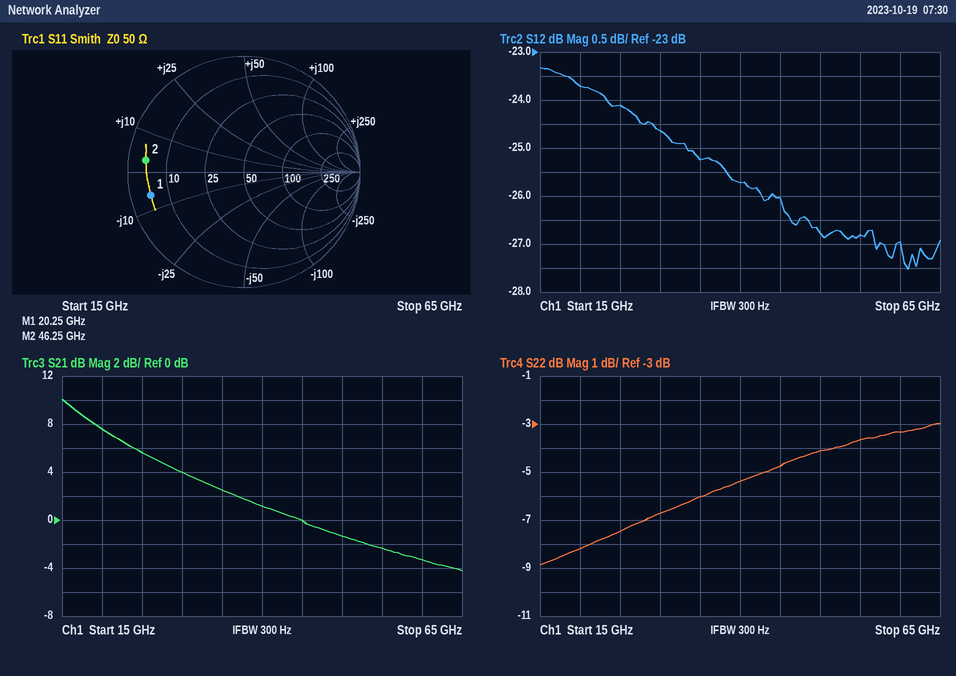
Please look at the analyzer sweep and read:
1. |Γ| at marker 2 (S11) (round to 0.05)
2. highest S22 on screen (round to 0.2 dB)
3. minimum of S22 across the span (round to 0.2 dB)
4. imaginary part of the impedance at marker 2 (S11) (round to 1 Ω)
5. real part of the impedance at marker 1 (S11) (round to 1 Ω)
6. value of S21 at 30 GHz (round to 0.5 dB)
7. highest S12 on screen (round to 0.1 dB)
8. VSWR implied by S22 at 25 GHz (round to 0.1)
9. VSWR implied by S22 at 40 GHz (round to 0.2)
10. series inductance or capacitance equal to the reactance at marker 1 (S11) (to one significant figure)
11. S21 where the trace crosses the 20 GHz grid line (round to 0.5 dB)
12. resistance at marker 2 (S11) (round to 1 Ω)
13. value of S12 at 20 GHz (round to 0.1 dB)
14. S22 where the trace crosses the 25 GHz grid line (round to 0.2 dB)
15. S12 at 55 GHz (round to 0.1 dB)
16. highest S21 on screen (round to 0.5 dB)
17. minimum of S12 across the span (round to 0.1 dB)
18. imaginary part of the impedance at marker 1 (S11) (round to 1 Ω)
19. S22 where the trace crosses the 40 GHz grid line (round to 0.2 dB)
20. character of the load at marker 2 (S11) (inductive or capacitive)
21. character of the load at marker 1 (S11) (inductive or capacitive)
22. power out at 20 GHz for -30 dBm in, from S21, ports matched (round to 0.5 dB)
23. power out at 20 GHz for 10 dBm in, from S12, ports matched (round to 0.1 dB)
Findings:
0.85
-3.0 dB
-8.8 dB
+3 Ω
5 Ω
4.0 dB
-23.3 dB
2.5
3.4
1 pF
7.5 dB
4 Ω
-23.7 dB
-7.4 dB
-26.8 dB
10.0 dB
-27.5 dB
-6 Ω
-5.4 dB
inductive
capacitive
-22.5 dBm
-13.7 dBm
